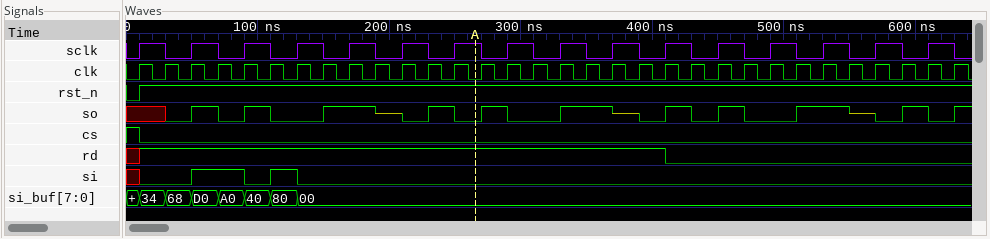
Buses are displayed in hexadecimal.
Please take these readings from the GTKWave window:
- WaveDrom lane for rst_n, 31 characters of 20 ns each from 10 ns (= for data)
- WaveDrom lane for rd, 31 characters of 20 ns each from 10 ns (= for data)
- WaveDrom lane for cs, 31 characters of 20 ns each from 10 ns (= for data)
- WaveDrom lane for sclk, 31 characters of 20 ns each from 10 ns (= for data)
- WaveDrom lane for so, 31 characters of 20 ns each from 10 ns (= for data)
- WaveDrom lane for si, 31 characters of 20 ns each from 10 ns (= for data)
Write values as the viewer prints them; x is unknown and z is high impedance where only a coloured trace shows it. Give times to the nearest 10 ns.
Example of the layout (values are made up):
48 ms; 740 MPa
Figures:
{name: 'rst_n', wave: '1..............................'}; {name: 'rd', wave: '1...................0..........'}; {name: 'cs', wave: '0..............................'}; {name: 'sclk', wave: '1010101010101010101010101010101'}; {name: 'so', wave: 'x01010.1.z01010.1.z01010.1.z010'}; {name: 'si', wave: '0.1.010........................'}
